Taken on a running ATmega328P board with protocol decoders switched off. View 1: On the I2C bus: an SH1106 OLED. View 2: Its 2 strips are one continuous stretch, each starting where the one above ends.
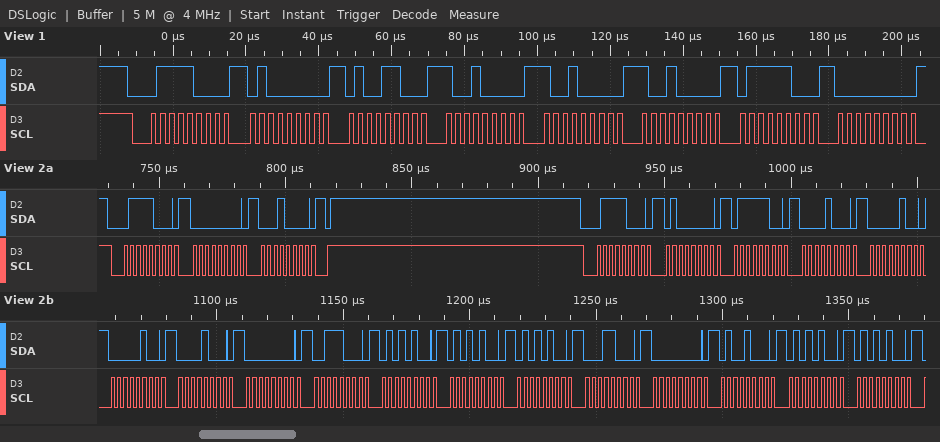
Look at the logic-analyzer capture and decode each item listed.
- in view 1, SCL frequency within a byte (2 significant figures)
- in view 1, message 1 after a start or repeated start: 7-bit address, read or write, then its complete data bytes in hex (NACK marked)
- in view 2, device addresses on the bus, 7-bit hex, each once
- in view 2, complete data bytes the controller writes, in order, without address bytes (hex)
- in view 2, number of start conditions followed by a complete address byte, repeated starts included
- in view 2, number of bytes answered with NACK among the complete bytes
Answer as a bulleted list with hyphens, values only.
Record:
- 400 kHz
- 0x3C write: 40 4C 90 90 90 7C 00
- 0x3C
- 00 10 40 7C 08 04 04 08 00 38 54 54 54 18 00 48 54 54
- 2
- 0
